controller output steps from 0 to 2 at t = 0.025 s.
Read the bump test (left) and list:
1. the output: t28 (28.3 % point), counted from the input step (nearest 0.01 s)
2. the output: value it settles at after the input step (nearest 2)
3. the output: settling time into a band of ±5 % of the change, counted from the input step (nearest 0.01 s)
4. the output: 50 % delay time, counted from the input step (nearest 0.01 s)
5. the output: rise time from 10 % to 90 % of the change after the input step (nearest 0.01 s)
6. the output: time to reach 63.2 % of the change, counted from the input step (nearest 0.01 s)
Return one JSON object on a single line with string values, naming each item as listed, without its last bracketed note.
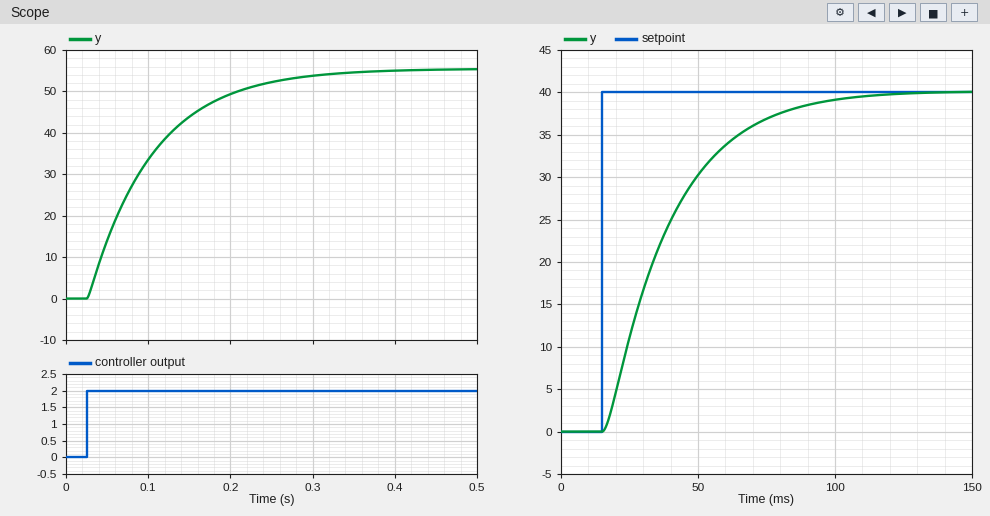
{"the output: t28 (28.3 % point), counted from the input step": "0.03 s", "the output: value it settles at after the input step": "56", "the output: settling time into a band of ±5 % of the change, counted from the input step": "0.24 s", "the output: 50 % delay time, counted from the input step": "0.06 s", "the output: rise time from 10 % to 90 % of the change after the input step": "0.17 s", "the output: time to reach 63.2 % of the change, counted from the input step": "0.08 s"}
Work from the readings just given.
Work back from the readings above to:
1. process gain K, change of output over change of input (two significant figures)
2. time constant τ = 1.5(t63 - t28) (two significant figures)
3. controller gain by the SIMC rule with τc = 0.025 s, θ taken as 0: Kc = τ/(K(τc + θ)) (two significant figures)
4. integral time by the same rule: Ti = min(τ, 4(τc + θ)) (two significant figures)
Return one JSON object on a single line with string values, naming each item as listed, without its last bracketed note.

{"process gain K, change of output over change of input": "28", "time constant τ = 1.5(t63 - t28)": "0.075 s", "controller gain by the SIMC rule with τc = 0.025 s, θ taken as 0: Kc = τ/(K(τc + θ))": "0.11", "integral time by the same rule: Ti = min(τ, 4(τc + θ))": "0.075 s"}
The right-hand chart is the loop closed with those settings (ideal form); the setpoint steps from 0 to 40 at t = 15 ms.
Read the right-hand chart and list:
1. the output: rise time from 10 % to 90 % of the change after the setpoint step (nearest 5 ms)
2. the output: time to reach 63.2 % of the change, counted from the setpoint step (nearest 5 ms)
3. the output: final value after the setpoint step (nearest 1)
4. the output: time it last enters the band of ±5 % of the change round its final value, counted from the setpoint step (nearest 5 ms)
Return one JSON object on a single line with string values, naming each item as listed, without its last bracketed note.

{"the output: rise time from 10 % to 90 % of the change after the setpoint step": "50 ms", "the output: time to reach 63.2 % of the change, counted from the setpoint step": "25 ms", "the output: final value after the setpoint step": "40", "the output: time it last enters the band of ±5 % of the change round its final value, counted from the setpoint step": "70 ms"}
